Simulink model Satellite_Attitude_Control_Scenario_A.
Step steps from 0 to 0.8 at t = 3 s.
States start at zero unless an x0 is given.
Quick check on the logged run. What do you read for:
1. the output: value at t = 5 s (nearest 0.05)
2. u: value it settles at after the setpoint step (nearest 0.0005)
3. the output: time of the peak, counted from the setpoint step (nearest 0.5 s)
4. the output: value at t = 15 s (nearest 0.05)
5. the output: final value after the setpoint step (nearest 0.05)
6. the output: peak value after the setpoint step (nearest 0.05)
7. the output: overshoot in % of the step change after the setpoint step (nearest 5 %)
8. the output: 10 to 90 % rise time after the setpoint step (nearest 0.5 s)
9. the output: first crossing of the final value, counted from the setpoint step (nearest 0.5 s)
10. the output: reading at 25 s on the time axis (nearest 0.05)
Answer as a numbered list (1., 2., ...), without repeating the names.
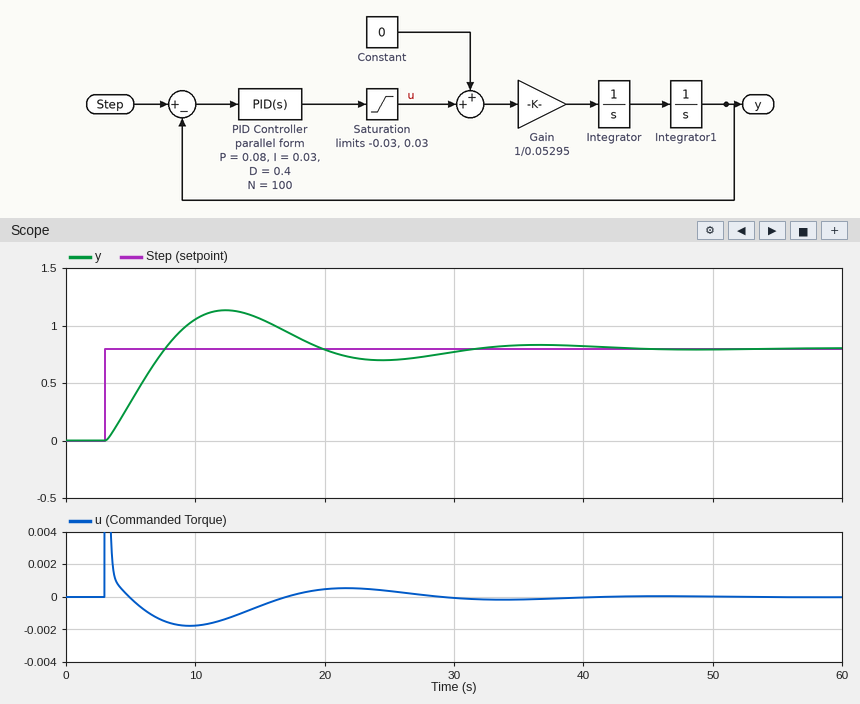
1. 0.35
2. 0.0000
3. 9.5 s
4. 1.05
5. 0.80
6. 1.15
7. 40 %
8. 3.5 s
9. 4.5 s
10. 0.70
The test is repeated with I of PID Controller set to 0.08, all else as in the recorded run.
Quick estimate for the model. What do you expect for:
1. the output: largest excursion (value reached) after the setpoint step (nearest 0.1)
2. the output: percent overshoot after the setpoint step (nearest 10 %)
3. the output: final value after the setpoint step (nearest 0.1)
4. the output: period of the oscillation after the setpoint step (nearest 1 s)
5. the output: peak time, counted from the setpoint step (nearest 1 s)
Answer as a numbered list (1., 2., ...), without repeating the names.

1. 1.3
2. 60 %
3. 0.8
4. 14 s
5. 6 s
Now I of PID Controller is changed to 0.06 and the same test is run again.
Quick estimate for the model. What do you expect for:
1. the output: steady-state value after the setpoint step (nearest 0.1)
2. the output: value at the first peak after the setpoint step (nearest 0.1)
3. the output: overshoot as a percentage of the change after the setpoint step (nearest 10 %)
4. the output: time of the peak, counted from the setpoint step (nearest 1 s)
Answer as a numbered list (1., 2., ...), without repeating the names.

1. 0.8
2. 1.2
3. 50 %
4. 7 s
